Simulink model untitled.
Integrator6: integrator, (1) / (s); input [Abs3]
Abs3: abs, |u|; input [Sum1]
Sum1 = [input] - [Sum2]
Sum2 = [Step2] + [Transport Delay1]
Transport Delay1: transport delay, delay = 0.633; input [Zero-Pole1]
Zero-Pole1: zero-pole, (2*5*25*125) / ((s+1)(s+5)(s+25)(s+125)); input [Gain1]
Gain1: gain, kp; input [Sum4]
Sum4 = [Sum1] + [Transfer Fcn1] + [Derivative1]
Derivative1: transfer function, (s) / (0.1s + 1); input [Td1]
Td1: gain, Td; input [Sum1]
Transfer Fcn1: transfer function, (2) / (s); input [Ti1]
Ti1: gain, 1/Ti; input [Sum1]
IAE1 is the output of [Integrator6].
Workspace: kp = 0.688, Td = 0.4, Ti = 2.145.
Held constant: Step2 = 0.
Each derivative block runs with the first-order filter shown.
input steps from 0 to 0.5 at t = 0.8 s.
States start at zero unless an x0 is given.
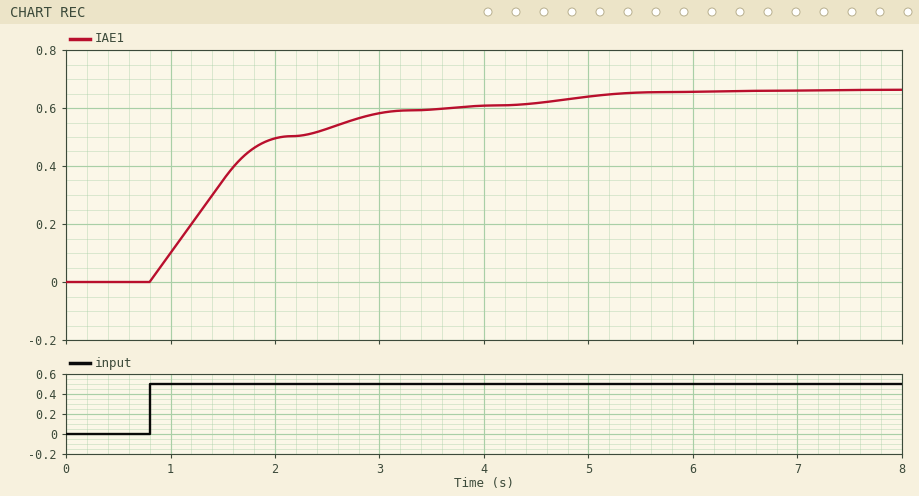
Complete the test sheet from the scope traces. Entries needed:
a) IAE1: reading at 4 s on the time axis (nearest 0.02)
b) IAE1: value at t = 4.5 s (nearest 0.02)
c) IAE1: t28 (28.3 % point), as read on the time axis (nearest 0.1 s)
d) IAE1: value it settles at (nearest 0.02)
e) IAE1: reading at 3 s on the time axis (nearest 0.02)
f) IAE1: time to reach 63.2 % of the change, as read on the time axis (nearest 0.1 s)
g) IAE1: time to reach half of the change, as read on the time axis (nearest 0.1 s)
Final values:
0.60
0.62
1.2 s
0.66
0.58
1.7 s
1.5 s
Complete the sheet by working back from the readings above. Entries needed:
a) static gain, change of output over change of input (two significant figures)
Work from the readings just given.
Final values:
1.3
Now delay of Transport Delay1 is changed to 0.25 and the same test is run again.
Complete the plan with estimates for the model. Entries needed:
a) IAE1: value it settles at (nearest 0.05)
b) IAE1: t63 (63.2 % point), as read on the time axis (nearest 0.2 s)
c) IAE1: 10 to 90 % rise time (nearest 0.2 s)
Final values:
0.45
1.4 s
1.8 s
